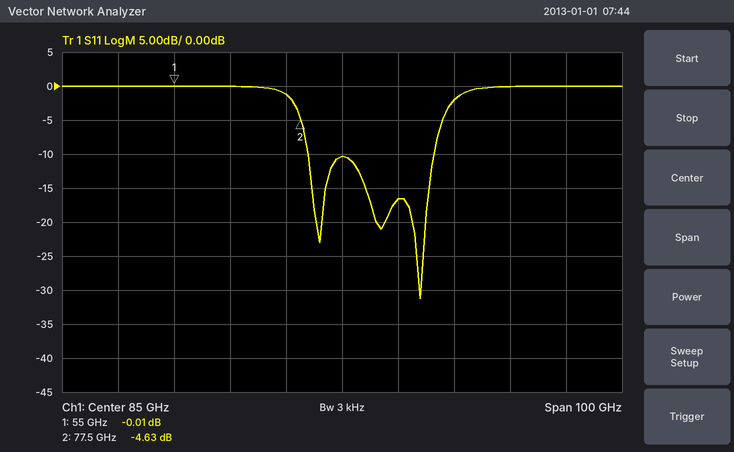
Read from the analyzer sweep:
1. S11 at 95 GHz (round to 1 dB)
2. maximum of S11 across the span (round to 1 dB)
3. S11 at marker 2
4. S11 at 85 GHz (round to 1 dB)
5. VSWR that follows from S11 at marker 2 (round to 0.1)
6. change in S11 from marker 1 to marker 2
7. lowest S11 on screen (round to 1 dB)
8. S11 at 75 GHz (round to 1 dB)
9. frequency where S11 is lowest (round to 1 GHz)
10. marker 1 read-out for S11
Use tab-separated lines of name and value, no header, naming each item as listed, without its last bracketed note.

S11 at 95 GHz	-17 dB
maximum of S11 across the span	0 dB
S11 at marker 2	-4.63 dB
S11 at 85 GHz	-10 dB
VSWR that follows from S11 at marker 2	3.8
change in S11 from marker 1 to marker 2	-4.62 dB
lowest S11 on screen	-31 dB
S11 at 75 GHz	-1 dB
frequency where S11 is lowest	99 GHz
marker 1 read-out for S11	-0.01 dB
